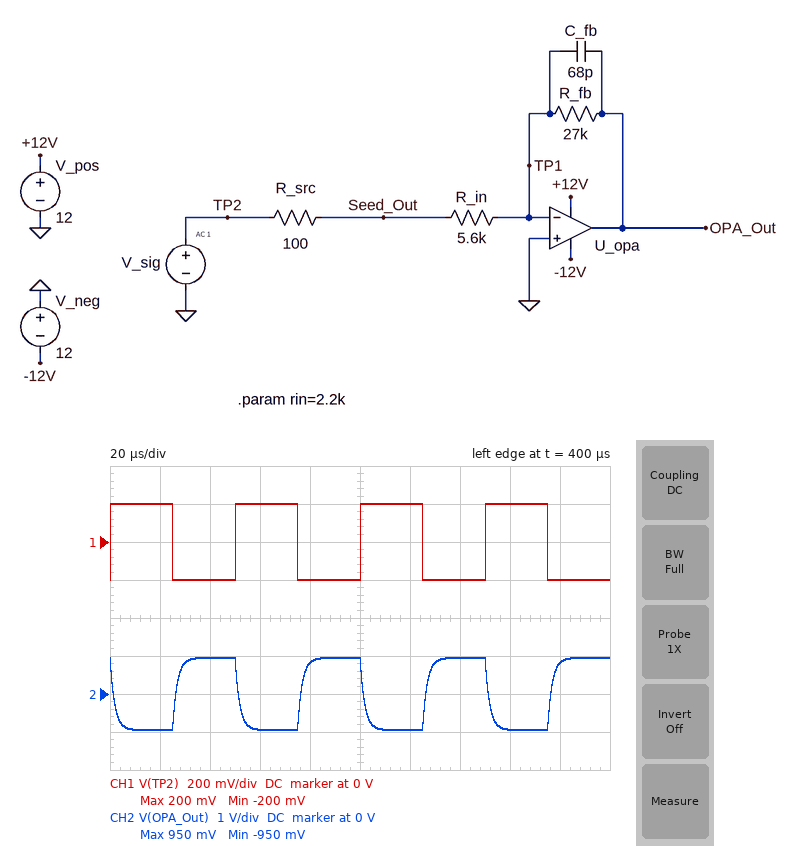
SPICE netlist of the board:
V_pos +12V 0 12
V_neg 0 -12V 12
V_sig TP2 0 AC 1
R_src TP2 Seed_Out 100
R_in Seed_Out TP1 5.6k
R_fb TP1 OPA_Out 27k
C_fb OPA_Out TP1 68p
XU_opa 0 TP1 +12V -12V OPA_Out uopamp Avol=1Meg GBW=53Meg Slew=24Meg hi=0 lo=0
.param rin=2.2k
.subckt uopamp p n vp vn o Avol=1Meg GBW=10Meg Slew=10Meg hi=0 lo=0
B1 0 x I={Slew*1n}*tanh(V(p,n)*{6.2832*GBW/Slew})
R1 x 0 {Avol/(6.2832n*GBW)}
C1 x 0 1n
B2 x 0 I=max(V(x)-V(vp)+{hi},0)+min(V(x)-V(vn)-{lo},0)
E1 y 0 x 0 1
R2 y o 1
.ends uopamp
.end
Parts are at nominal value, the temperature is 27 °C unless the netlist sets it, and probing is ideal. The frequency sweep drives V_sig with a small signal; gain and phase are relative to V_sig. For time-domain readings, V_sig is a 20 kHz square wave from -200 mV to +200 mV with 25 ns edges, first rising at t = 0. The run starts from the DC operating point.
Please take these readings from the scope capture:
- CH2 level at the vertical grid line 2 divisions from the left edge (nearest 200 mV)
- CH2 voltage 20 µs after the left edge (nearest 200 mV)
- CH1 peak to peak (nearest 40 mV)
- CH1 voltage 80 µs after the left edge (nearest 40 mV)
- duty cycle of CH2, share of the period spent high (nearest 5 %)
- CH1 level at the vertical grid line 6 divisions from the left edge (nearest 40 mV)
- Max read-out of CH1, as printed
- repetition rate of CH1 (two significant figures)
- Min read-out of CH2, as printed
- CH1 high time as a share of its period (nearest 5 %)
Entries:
1.0 V
-1.0 V
400 mV
-200 mV
50 %
200 mV
200 mV
20 kHz
-950 mV
50 %
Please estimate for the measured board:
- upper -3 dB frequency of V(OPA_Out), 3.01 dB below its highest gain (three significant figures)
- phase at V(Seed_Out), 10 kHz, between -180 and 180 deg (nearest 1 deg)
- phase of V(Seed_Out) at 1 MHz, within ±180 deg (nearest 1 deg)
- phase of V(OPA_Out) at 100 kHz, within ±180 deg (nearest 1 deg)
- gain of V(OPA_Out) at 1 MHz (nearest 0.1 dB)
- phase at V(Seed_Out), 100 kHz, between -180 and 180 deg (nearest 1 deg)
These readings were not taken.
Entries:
86.0 kHz
0 deg
0 deg
131 deg
-7.8 dB
0 deg
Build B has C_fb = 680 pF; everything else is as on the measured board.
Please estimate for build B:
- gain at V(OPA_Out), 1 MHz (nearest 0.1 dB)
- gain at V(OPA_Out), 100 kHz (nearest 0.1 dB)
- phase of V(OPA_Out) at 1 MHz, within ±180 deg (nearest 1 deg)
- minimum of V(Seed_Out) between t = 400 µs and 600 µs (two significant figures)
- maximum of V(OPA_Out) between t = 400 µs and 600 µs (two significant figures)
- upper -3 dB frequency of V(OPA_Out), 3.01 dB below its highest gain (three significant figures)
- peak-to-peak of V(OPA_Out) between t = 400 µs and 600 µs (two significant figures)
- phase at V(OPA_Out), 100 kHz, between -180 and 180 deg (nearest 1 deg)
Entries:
-27.7 dB
-7.8 dB
89 deg
-200 mV
560 mV
8.66 kHz
1.1 V
95 deg
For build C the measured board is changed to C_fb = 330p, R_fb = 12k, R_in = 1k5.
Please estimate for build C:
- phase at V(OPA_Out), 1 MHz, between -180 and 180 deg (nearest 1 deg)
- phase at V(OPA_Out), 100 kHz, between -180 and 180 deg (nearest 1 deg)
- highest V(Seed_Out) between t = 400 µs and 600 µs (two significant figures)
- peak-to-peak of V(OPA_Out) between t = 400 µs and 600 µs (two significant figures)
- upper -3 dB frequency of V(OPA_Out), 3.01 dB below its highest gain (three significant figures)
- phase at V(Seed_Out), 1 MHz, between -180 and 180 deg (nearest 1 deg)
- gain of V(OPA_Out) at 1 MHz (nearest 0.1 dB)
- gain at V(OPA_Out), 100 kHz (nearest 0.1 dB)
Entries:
91 deg
112 deg
190 mV
3.0 V
40.0 kHz
0 deg
-10.5 dB
8.9 dB
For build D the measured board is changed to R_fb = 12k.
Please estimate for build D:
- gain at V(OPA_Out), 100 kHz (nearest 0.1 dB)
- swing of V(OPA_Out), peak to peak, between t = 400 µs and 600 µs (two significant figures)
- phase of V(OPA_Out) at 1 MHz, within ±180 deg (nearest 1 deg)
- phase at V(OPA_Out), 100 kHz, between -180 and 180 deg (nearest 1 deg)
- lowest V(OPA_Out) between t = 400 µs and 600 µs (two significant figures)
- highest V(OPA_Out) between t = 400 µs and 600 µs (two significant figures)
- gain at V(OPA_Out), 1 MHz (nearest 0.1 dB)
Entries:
5.4 dB
840 mV
100 deg
153 deg
-420 mV
420 mV
-8.0 dB
